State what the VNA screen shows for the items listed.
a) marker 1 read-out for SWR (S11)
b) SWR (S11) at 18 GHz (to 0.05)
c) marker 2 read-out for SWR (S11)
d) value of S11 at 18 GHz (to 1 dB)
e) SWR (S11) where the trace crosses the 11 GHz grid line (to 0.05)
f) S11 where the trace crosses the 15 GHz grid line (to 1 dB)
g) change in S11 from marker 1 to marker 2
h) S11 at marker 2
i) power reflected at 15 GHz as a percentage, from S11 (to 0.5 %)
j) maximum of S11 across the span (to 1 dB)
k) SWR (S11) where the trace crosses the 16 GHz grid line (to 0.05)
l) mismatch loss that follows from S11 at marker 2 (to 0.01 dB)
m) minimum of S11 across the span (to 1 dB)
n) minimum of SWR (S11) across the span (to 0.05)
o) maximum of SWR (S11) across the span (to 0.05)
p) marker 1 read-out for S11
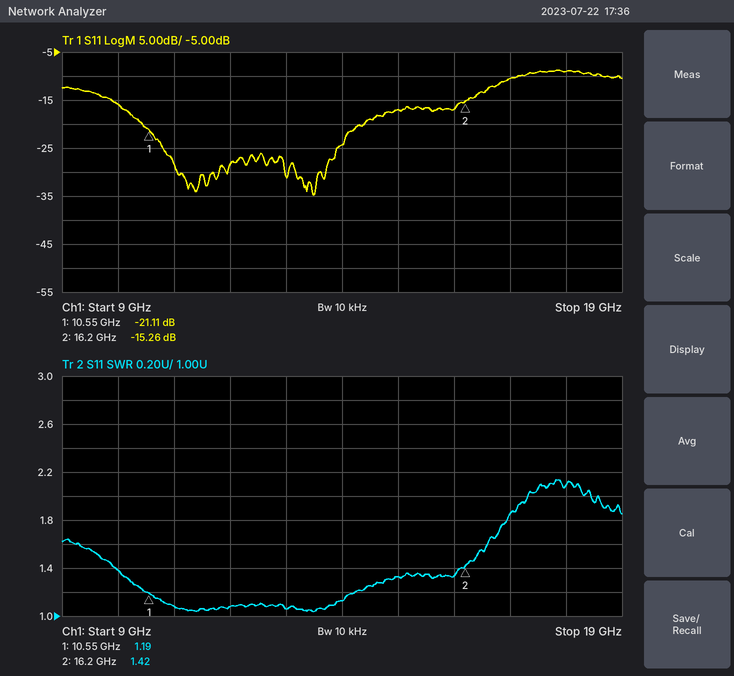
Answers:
1.19
2.10
1.42
-9 dB
1.10
-17 dB
5.85 dB
-15.26 dB
2.0 %
-9 dB
1.35
0.13 dB
-35 dB
1.05
2.15
-21.11 dB
